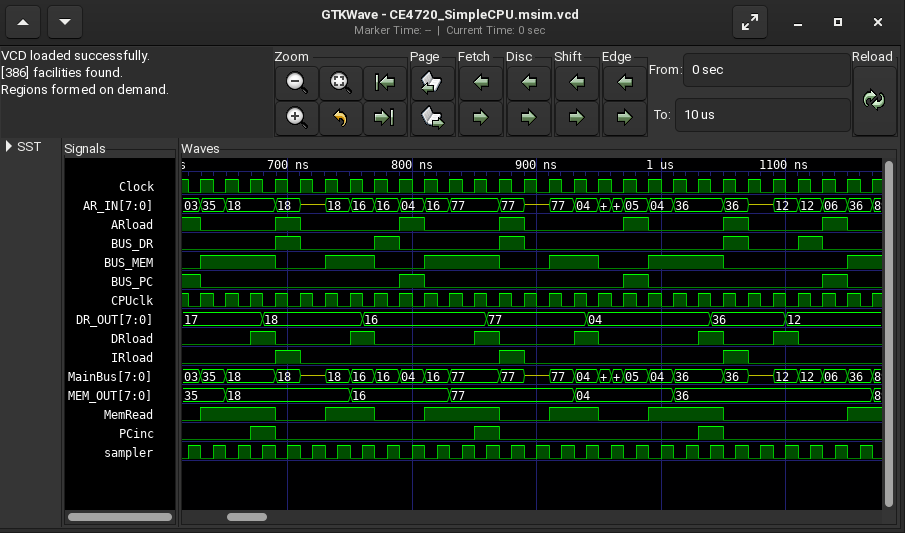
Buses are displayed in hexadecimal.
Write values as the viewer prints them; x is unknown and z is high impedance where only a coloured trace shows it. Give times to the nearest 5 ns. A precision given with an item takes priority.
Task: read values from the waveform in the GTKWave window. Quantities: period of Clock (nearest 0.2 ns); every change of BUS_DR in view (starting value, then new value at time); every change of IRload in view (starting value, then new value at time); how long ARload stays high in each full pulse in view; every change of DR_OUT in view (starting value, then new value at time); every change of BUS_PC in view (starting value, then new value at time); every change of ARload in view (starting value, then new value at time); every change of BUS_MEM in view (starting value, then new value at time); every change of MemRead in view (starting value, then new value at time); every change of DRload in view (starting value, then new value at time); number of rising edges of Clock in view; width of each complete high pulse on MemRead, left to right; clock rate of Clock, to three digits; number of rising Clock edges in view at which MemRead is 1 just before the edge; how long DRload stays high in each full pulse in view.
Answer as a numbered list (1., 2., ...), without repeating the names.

1. 20 ns
2. 0, 1 at 690 ns, 0 at 710 ns, 1 at 770 ns, 0 at 790 ns, 1 at 870 ns, 0 at 890 ns, 1 at 1050 ns, 0 at 1070 ns, 1 at 1110 ns, 0 at 1130 ns
3. 0, 1 at 690 ns, 0 at 710 ns, 1 at 870 ns, 0 at 890 ns, 1 at 1050 ns, 0 at 1070 ns
4. 20 ns, 20 ns, 20 ns, 20 ns, 20 ns, 20 ns
5. 17, 18 at 680 ns, 16 at 760 ns, 77 at 860 ns, 04 at 940 ns, 36 at 1040 ns, 12 at 1100 ns
6. 1, 0 at 630 ns, 1 at 790 ns, 0 at 810 ns, 1 at 970 ns, 0 at 990 ns, 1 at 1130 ns, 0 at 1150 ns
7. 1, 0 at 630 ns, 1 at 690 ns, 0 at 710 ns, 1 at 790 ns, 0 at 810 ns, 1 at 870 ns, 0 at 890 ns, 1 at 970 ns, 0 at 990 ns, 1 at 1050 ns, 0 at 1070 ns, 1 at 1130 ns, 0 at 1150 ns
8. 0, 1 at 630 ns, 0 at 690 ns, 1 at 730 ns, 0 at 770 ns, 1 at 810 ns, 0 at 870 ns, 1 at 910 ns, 0 at 950 ns, 1 at 990 ns, 0 at 1050 ns, 1 at 1150 ns
9. 0, 1 at 630 ns, 0 at 690 ns, 1 at 730 ns, 0 at 770 ns, 1 at 810 ns, 0 at 870 ns, 1 at 910 ns, 0 at 950 ns, 1 at 990 ns, 0 at 1050 ns, 1 at 1150 ns
10. 0, 1 at 670 ns, 0 at 690 ns, 1 at 750 ns, 0 at 770 ns, 1 at 850 ns, 0 at 870 ns, 1 at 930 ns, 0 at 950 ns, 1 at 1030 ns, 0 at 1050 ns, 1 at 1090 ns, 0 at 1110 ns
11. 28
12. 60 ns, 40 ns, 60 ns, 40 ns, 60 ns
13. 50.0 MHz
14. 14
15. 20 ns, 20 ns, 20 ns, 20 ns, 20 ns, 20 ns
